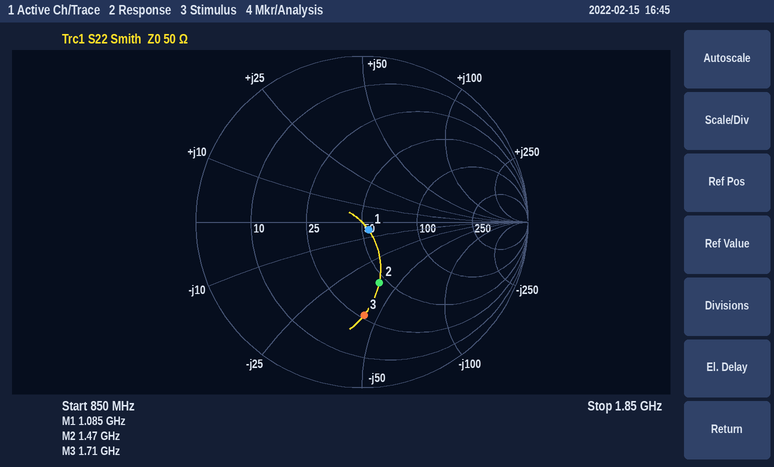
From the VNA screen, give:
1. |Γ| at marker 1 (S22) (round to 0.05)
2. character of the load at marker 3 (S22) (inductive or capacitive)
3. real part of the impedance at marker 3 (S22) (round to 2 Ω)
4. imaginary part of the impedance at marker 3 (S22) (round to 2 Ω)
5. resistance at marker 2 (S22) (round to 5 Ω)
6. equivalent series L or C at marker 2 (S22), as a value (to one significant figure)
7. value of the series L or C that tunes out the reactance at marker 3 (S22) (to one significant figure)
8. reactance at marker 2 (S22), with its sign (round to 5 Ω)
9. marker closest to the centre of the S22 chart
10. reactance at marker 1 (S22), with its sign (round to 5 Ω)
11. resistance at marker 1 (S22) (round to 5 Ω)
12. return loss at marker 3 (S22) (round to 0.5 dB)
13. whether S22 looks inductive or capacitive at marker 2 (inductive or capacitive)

0.05
capacitive
26 Ω
-44 Ω
45 Ω
3 pF
4 nH
-40 Ω
marker 1
-5 Ω
55 Ω
5.0 dB
capacitive
